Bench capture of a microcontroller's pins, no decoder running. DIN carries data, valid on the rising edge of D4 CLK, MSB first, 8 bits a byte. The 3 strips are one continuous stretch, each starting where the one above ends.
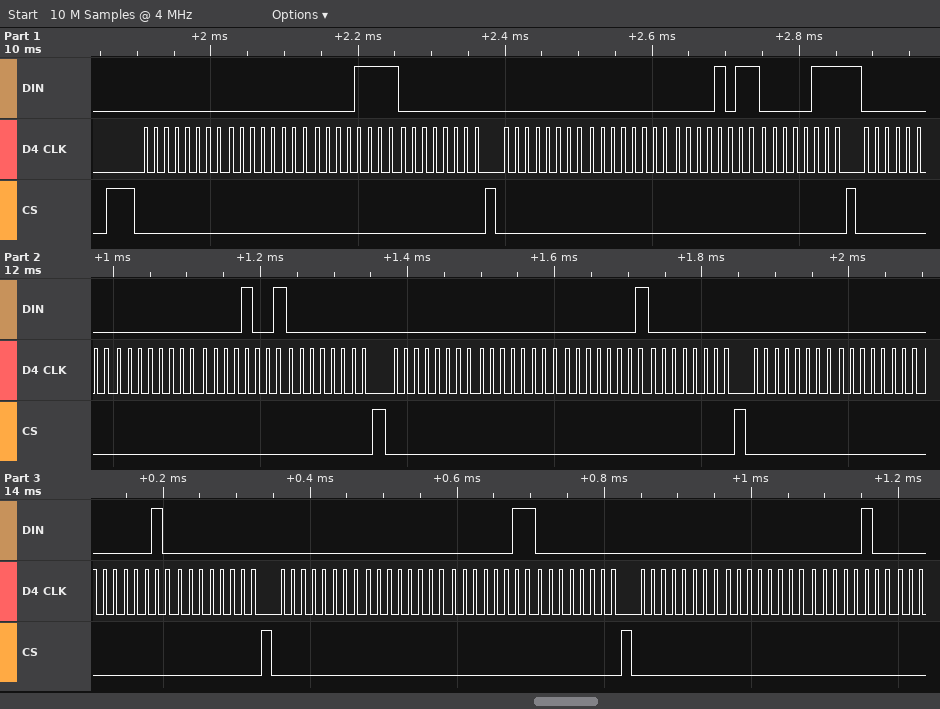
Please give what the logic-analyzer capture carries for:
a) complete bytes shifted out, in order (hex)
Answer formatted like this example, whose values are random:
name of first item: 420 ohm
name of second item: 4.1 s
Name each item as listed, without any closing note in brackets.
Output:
complete bytes shifted out, in order: 0x00 0x00 0x0F 0x00 0x00 0x00 0x0B 0x07 0x00 0x00 0x09 0x00 0x00 0x00 0x01 0x00 0x00 0x00 0x02 0x00 0x00 0x00 0x03 0x00 0x00 0x00 0x04
